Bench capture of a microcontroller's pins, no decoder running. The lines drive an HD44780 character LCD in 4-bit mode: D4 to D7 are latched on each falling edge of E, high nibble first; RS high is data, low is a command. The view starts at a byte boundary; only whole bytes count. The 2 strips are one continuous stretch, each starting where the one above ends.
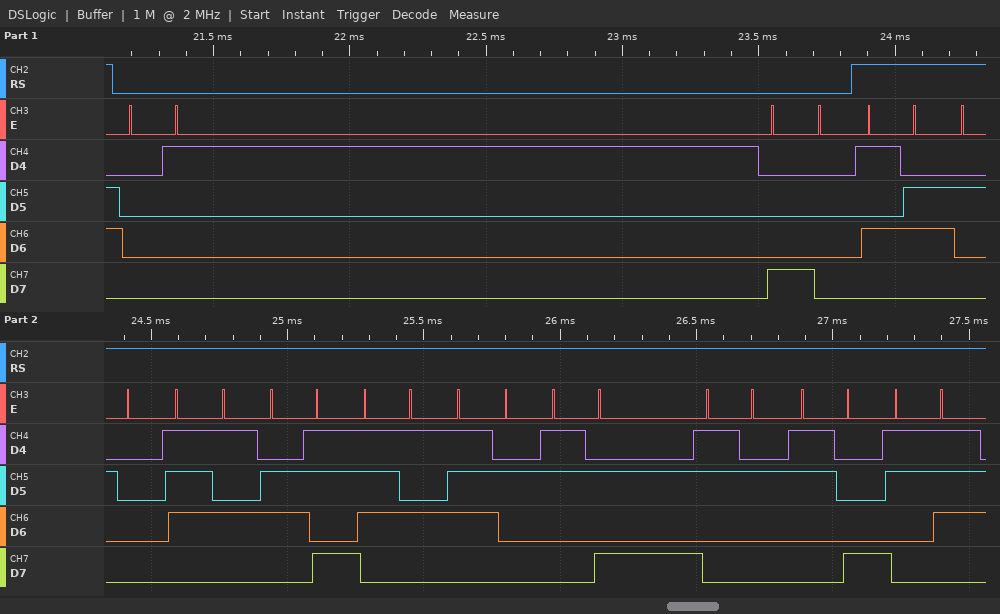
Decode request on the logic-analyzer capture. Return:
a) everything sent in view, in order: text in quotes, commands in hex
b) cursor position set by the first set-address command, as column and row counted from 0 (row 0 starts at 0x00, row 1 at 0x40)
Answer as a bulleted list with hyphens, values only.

- 0x01 0x80 "V ukur:287"
- column 0, row 0
